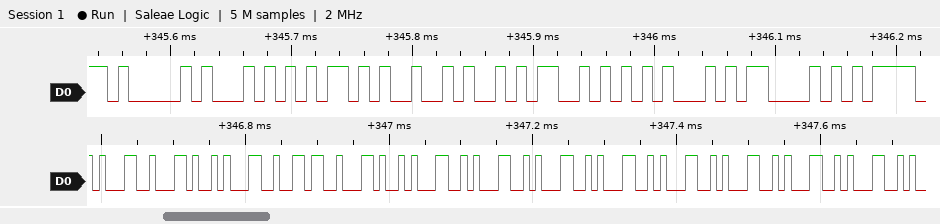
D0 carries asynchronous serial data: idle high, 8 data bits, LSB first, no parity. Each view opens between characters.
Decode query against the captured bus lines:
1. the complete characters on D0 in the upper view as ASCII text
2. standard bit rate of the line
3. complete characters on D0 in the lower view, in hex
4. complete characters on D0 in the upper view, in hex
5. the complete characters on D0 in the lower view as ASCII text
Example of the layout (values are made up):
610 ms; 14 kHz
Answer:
"AT+JSEC"; 115200 baud; 31, 2C, 31, 36, 2C, 31, 31, 31, 31, 31, 31, 31, 31; 41, 54, 2B, 4A, 53, 45, 43; "1,16,11111111"
